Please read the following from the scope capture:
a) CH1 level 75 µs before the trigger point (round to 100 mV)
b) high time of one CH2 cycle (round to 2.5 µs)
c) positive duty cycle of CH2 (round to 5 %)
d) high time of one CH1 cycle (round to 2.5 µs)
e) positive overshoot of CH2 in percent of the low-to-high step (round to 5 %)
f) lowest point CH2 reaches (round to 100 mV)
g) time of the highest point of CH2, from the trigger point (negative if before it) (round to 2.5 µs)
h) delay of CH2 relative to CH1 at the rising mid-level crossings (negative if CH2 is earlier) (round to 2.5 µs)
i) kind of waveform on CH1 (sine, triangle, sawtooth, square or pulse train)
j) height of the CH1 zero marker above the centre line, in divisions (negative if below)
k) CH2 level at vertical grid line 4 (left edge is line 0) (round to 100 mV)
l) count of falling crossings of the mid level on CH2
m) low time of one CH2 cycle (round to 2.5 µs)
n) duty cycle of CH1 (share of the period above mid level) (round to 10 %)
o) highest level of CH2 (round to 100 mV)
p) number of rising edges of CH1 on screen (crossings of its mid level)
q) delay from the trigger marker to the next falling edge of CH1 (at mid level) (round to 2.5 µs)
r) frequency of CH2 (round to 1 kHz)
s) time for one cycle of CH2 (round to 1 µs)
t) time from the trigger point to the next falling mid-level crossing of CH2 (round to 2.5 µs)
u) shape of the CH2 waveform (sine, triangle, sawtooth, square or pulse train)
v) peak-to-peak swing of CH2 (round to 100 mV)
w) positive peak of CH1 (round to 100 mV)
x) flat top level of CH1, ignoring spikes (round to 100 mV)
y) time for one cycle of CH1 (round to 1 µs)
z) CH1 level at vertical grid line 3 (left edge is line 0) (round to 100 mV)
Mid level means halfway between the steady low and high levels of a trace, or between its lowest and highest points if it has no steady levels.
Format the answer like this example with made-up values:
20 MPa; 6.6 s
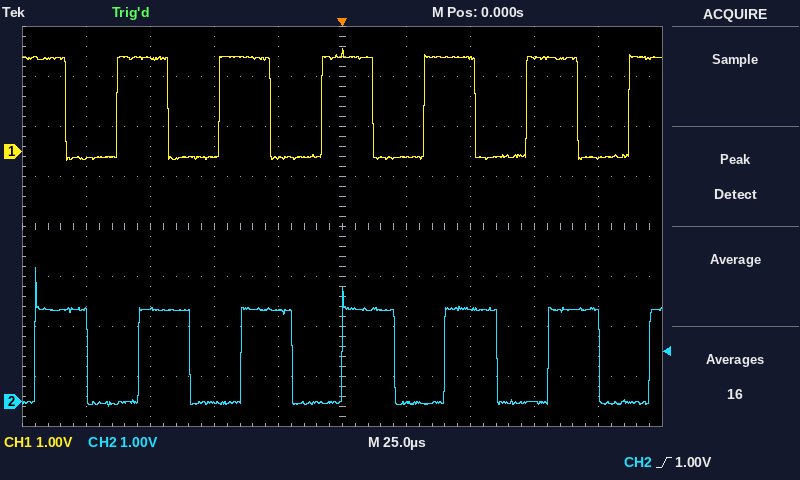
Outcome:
1.9 V; 20.0 µs; 50 %; 20.0 µs; 45 %; -100 mV; -120.0 µs; +7.5 µs; square; +1.5 div; 1.8 V; 6; 20.0 µs; 50 %; 2.7 V; 6; 12.5 µs; 25 kHz; 40 µs; 20.0 µs; square; 2.8 V; 2.1 V; 1.9 V; 40 µs; -100 mV
